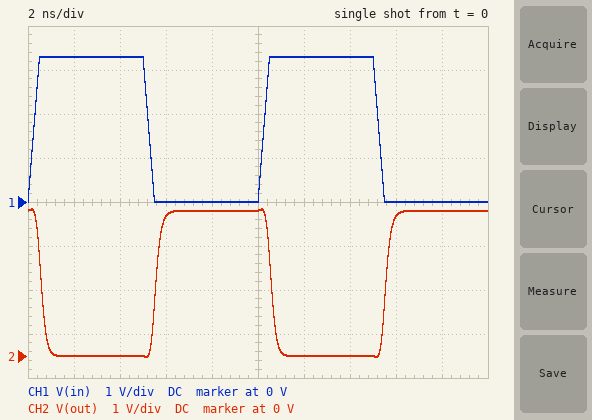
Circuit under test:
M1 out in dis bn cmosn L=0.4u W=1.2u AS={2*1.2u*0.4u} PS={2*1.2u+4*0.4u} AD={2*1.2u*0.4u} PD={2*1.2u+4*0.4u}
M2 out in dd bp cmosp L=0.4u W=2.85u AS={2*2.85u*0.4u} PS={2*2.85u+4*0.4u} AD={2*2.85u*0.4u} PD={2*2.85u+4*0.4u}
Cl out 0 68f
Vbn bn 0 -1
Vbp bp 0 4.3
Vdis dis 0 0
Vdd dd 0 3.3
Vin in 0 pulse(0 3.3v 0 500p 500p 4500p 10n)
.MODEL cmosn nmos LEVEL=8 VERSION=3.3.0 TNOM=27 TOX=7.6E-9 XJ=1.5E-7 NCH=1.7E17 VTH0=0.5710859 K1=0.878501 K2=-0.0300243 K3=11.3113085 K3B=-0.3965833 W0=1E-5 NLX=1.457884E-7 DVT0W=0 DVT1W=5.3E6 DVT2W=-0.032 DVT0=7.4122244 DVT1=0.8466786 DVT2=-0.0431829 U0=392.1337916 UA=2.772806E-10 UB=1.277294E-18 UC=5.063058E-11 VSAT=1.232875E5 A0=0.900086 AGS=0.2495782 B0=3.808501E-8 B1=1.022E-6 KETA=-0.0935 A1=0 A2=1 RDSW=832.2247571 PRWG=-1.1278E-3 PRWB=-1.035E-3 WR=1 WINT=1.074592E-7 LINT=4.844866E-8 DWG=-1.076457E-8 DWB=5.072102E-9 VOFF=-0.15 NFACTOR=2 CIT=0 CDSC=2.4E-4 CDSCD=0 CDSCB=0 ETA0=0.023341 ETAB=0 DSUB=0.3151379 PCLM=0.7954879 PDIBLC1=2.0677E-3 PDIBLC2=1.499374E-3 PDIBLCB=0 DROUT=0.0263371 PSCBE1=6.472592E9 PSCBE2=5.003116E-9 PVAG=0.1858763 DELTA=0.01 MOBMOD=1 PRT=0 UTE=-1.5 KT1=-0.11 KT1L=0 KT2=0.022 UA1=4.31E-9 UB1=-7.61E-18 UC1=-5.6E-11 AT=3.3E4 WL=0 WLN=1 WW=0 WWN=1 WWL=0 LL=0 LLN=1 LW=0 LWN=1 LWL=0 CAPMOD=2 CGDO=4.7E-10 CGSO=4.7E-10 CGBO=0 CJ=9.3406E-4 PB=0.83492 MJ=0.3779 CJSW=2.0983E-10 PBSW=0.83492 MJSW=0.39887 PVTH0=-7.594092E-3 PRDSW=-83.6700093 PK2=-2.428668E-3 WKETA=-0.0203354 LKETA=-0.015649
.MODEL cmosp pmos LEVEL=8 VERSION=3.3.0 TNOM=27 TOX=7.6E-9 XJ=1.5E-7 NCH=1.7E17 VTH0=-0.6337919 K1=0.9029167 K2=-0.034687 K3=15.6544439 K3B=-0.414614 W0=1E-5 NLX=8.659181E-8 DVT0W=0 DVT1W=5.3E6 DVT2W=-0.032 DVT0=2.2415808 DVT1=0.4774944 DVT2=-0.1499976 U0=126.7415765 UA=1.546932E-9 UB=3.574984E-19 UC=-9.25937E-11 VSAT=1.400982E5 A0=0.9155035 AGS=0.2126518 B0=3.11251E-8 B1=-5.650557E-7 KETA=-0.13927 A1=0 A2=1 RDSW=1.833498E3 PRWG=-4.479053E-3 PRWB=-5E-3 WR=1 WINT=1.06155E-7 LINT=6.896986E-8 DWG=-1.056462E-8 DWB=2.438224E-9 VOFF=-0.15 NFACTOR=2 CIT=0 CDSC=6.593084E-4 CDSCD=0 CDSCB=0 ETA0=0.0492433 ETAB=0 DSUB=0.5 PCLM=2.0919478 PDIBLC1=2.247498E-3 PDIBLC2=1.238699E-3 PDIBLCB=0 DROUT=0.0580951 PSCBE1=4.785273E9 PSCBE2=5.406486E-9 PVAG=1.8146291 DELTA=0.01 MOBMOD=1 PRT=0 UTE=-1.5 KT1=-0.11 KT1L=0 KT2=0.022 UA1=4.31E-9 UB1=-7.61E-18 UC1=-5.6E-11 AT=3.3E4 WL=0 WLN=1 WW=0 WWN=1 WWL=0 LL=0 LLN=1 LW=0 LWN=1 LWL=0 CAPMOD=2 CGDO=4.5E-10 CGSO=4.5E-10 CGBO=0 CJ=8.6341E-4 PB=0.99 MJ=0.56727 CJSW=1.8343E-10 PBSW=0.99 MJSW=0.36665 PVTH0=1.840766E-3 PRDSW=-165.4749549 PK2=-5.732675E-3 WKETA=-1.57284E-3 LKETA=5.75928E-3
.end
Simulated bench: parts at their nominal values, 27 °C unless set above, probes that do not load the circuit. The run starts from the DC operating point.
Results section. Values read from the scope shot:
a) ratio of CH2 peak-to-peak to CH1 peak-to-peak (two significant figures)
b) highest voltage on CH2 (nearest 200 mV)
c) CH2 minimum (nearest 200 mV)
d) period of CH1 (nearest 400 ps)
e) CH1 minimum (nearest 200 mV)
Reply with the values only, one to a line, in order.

1.0
3.4 V
0 V
10.0 ns
0 V
